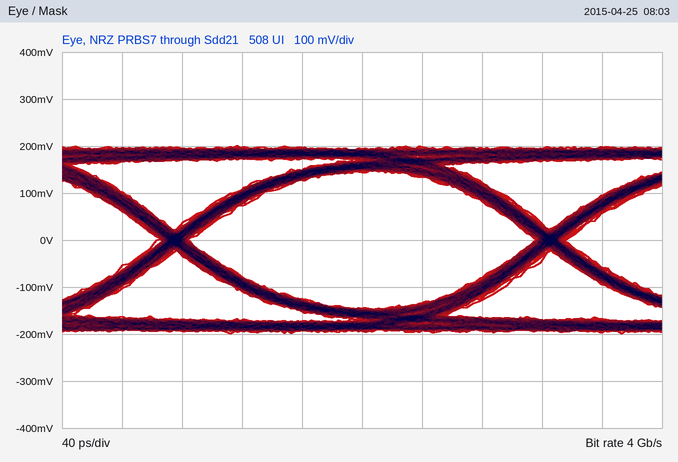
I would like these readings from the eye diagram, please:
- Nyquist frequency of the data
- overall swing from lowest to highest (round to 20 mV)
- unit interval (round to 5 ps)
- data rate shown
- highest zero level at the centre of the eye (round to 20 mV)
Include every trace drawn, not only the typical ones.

2 GHz
400 mV
250 ps
4 Gb/s
-140 mV
